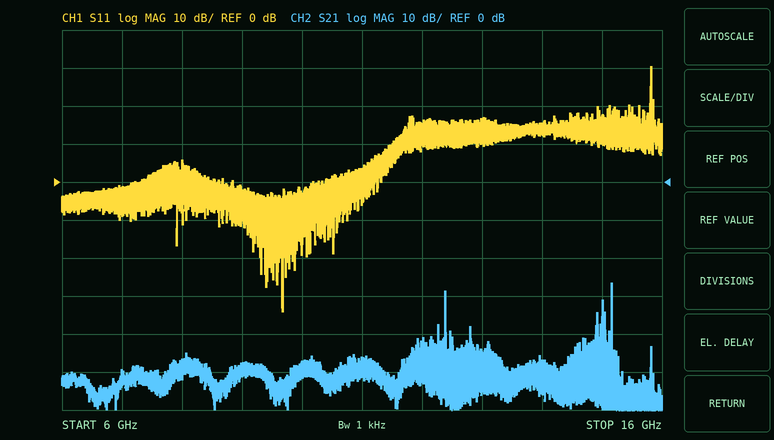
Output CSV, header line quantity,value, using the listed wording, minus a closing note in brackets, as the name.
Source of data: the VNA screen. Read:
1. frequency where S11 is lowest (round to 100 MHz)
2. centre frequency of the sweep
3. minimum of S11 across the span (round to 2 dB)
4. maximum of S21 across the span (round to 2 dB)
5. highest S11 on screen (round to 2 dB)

quantity,value
frequency where S11 is lowest,9.7 GHz
centre frequency of the sweep,11 GHz
minimum of S11 across the span,-34 dB
maximum of S21 across the span,-26 dB
highest S11 on screen,30 dB
